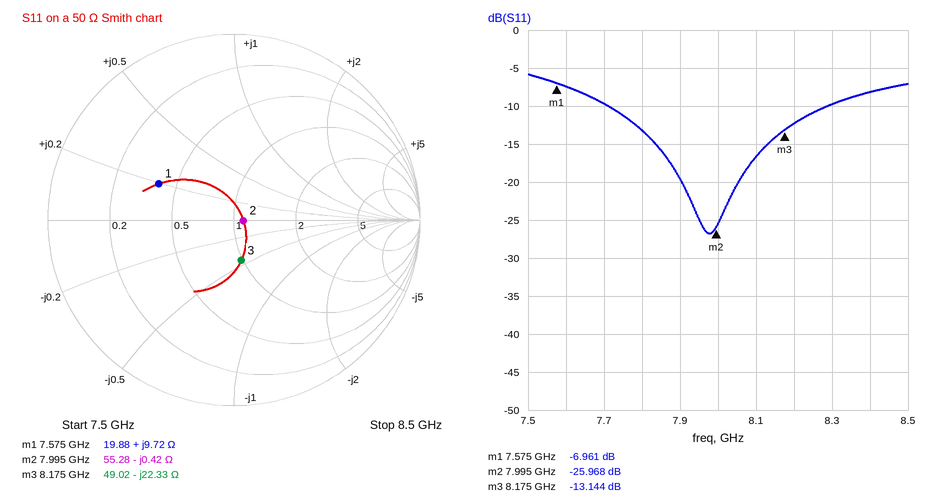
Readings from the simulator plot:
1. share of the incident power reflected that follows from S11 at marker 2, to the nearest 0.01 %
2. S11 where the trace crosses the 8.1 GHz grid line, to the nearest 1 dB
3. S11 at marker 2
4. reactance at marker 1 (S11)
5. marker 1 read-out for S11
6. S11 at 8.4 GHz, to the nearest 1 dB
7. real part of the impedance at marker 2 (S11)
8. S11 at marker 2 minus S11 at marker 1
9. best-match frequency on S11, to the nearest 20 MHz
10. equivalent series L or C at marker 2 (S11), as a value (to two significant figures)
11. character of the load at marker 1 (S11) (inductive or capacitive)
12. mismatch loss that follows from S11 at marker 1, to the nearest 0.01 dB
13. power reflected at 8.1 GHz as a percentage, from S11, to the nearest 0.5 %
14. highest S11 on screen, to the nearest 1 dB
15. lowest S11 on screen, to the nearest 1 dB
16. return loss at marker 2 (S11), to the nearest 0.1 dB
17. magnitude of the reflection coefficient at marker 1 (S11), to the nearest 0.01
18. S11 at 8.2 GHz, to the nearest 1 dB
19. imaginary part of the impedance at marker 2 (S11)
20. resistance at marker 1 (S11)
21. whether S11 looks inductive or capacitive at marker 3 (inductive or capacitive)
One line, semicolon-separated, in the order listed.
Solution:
0.25 %; -17 dB; -25.968 dB; +9.72 Ω; -6.961 dB; -8 dB; 55.28 Ω; -19.007 dB; 7.98 GHz; 47 pF; inductive; 0.98 dB; 2.0 %; -6 dB; -27 dB; 26.0 dB; 0.45; -12 dB; -0.42 Ω; 19.88 Ω; capacitive
